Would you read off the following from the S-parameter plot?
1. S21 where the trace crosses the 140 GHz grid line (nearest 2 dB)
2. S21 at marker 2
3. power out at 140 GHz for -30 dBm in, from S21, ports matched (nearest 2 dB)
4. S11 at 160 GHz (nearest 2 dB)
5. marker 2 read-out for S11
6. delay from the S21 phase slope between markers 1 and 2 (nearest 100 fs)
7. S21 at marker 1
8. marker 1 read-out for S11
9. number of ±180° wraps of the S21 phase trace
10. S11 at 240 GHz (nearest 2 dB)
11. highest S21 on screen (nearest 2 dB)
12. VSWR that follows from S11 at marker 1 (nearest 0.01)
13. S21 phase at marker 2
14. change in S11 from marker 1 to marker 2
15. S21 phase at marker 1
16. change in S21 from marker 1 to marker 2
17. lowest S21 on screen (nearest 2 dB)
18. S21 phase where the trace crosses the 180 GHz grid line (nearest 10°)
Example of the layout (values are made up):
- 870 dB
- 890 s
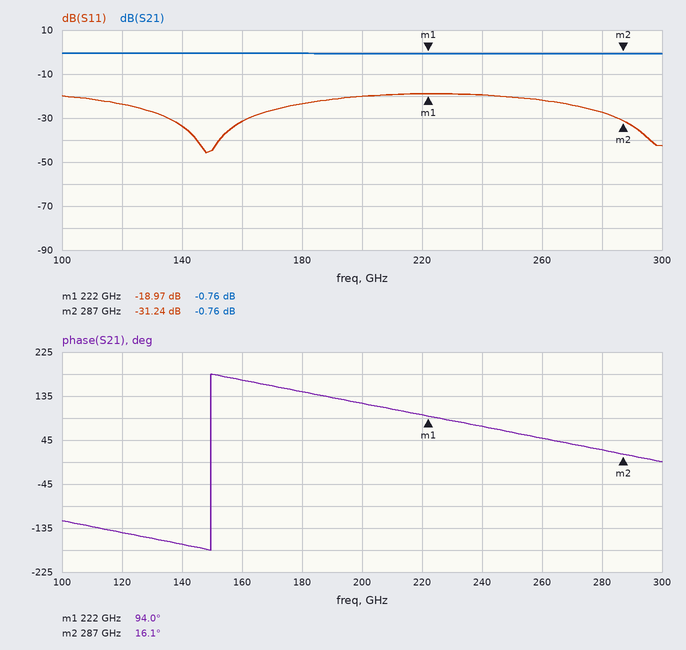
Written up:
- 0 dB
- -0.76 dB
- -30 dBm
- -32 dB
- -31.24 dB
- 3.3 ps
- -0.76 dB
- -18.97 dB
- 1
- -20 dB
- 0 dB
- 1.25
- 16.1°
- -12.27 dB
- 94.0°
- 0.00 dB
- 0 dB
- 140°
